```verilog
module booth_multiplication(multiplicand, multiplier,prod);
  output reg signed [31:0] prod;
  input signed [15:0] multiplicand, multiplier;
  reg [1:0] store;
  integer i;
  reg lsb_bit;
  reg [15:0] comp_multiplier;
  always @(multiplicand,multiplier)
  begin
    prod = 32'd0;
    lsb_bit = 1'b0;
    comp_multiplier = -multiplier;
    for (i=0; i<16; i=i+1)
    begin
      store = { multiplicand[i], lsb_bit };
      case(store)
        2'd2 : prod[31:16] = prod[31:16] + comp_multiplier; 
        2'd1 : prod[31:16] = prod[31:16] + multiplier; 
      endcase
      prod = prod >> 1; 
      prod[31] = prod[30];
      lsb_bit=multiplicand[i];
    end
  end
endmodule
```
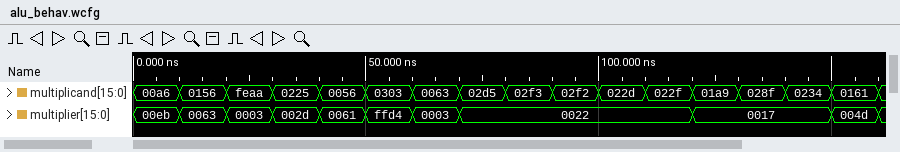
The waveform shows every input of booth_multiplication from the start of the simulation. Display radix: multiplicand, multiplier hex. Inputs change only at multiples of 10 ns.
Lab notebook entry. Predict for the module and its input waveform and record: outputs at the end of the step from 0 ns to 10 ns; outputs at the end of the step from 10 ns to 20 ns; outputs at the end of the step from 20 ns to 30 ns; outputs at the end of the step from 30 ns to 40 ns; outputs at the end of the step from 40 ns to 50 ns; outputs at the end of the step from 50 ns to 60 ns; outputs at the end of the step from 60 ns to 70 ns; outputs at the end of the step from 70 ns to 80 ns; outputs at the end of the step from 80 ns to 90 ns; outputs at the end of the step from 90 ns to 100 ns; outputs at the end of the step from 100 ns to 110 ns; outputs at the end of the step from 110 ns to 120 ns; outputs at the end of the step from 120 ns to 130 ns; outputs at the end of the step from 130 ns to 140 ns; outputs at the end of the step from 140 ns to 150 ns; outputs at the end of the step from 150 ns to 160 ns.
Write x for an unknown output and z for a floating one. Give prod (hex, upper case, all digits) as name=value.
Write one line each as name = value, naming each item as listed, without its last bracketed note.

outputs at the end of the step from 0 ns to 10 ns = prod=00009862
outputs at the end of the step from 10 ns to 20 ns = prod=00008442
outputs at the end of the step from 20 ns to 30 ns = prod=FFFFFBFE
outputs at the end of the step from 30 ns to 40 ns = prod=00006081
outputs at the end of the step from 40 ns to 50 ns = prod=00002096
outputs at the end of the step from 50 ns to 60 ns = prod=FFFF7B7C
outputs at the end of the step from 60 ns to 70 ns = prod=00000129
outputs at the end of the step from 70 ns to 80 ns = prod=0000604A
outputs at the end of the step from 80 ns to 90 ns = prod=00006446
outputs at the end of the step from 90 ns to 100 ns = prod=00006424
outputs at the end of the step from 100 ns to 110 ns = prod=000049FA
outputs at the end of the step from 110 ns to 120 ns = prod=00004A3E
outputs at the end of the step from 120 ns to 130 ns = prod=0000262F
outputs at the end of the step from 130 ns to 140 ns = prod=00003AD9
outputs at the end of the step from 140 ns to 150 ns = prod=000032AC
outputs at the end of the step from 150 ns to 160 ns = prod=00006A2D
